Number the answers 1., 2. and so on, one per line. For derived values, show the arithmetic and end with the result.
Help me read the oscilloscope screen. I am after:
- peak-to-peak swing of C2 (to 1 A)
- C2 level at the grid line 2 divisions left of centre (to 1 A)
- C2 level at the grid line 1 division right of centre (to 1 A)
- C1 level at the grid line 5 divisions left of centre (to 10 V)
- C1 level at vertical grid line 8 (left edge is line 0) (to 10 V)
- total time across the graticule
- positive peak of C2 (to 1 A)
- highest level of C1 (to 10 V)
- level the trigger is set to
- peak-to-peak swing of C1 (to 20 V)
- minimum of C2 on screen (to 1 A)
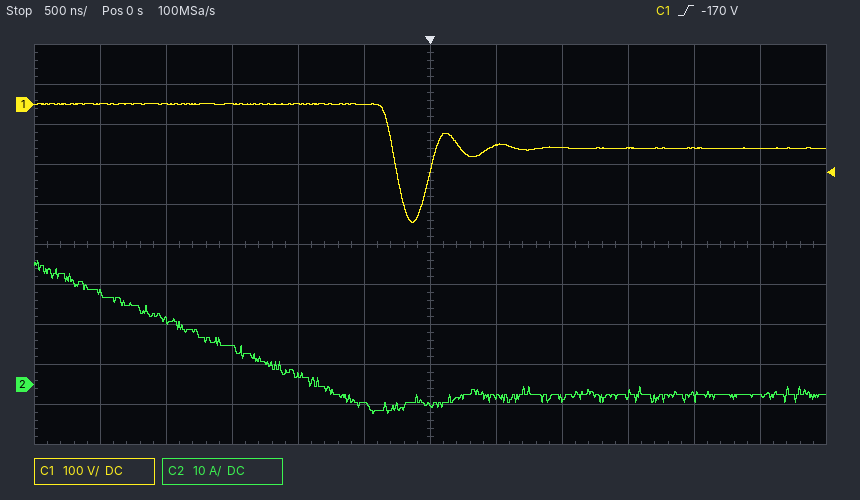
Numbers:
1. 31 A − (-7 A) = 38 A
2. 2 A
3. -3 A
4. 0 V
5. -110 V
6. 6 µs
7. 31 A
8. 0 V
9. -170 V
10. 300 V
11. -7 A
